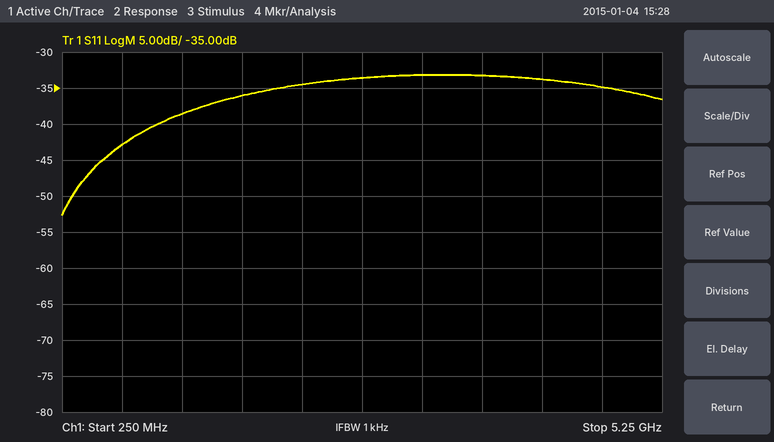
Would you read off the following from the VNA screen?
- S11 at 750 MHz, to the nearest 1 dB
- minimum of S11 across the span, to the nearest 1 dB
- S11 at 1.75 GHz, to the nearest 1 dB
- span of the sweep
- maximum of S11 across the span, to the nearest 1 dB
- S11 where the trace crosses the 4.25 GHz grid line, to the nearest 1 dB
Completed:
-43 dB
-53 dB
-36 dB
5 GHz
-33 dB
-34 dB
